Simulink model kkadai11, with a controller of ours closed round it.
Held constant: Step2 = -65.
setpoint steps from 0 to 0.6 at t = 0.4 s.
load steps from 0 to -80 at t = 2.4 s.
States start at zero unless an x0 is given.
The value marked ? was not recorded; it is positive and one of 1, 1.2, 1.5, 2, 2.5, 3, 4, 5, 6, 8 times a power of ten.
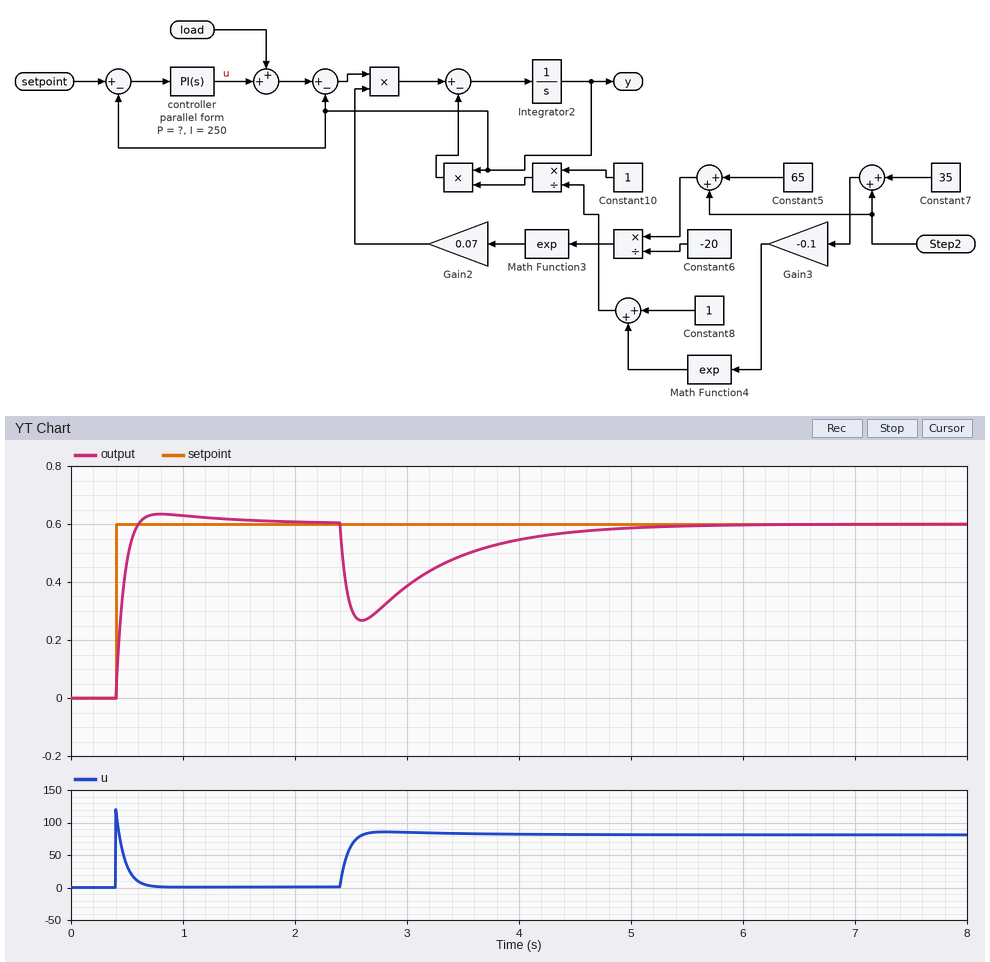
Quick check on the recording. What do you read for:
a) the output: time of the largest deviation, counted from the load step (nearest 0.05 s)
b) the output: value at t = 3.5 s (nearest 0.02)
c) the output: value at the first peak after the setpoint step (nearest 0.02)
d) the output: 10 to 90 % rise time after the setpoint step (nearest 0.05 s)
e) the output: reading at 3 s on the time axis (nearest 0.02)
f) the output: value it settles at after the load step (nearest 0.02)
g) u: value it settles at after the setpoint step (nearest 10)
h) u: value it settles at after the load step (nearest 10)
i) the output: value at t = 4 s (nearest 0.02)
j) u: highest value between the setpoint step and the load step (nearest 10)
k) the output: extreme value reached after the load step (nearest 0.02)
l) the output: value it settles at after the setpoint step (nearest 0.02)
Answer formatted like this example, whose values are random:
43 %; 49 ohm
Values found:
0.20 s; 0.50; 0.64; 0.15 s; 0.38; 0.60; 0; 80; 0.54; 120; 0.26; 0.60
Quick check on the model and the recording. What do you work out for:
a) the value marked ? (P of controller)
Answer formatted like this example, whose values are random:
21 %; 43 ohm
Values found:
200
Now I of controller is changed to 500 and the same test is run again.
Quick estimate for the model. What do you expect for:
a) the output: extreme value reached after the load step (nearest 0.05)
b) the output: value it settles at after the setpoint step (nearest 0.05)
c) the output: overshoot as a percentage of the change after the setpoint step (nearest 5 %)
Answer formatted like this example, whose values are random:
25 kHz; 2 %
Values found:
0.30; 0.60; 10 %
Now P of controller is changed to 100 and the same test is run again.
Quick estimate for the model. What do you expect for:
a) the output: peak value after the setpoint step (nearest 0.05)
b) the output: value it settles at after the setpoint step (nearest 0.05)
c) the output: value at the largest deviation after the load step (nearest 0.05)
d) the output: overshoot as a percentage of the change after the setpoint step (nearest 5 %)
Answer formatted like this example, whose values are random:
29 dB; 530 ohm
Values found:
0.70; 0.60; 0.05; 15 %
